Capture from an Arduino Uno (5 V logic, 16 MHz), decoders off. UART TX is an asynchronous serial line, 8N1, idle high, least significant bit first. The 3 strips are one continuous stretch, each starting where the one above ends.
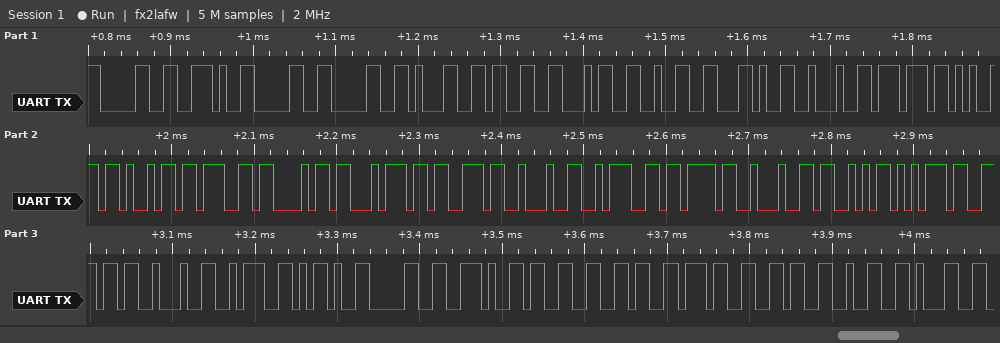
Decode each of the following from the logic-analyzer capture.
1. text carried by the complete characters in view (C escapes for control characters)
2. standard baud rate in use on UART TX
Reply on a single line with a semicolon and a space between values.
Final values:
"0.001342,\"weights\":{\"Sun\":-0.367621"; 115200 baud
